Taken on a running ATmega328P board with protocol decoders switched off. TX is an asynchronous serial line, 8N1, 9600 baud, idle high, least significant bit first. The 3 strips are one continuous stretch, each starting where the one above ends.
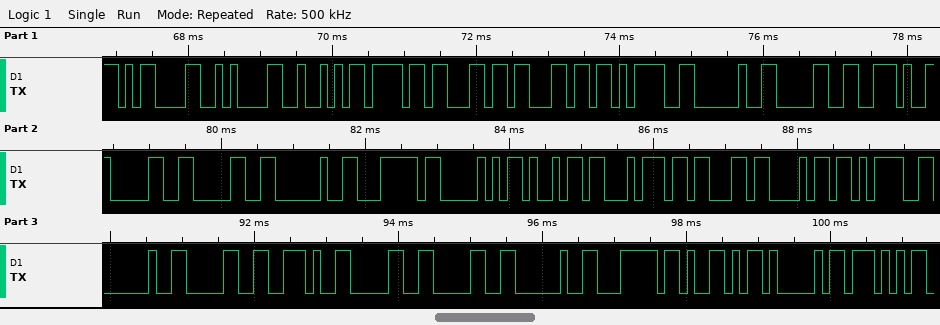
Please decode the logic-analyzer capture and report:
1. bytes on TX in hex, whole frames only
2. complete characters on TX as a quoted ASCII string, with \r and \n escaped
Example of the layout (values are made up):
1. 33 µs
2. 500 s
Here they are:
1. 0D 0A 52 6F 6C 6C 3D 20 30 2E 30 30 20 7C 50 69 74 63 68 3D 20 30 2E 30 30 20 7C 59 41 57
2. "\r\nRoll= 0.00 |Pitch= 0.00 |YAW"
